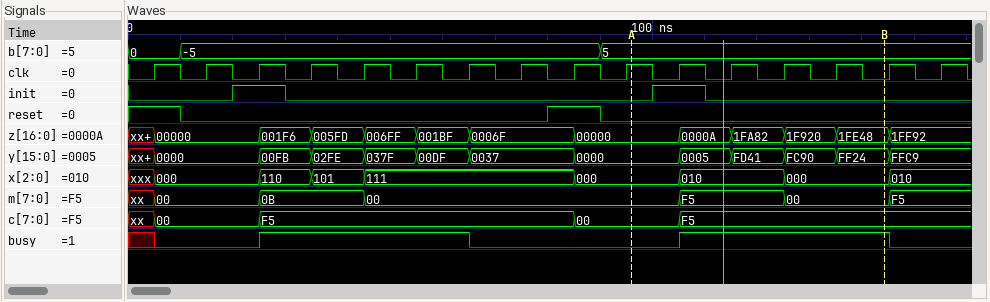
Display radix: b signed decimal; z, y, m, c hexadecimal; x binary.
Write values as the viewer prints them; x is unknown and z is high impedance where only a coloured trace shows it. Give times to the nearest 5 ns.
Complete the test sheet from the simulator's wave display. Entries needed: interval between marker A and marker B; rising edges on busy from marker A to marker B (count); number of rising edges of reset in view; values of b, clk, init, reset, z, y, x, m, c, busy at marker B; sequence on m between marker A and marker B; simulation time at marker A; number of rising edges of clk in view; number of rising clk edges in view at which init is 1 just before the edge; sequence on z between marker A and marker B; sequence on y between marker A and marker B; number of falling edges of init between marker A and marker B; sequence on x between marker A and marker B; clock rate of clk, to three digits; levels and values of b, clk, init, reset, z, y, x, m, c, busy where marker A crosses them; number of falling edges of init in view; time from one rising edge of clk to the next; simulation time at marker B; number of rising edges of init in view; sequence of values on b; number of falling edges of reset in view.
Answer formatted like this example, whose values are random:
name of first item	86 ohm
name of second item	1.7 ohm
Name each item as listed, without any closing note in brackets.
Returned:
interval between marker A and marker B	50 ns
rising edges on busy from marker A to marker B	1
number of rising edges of reset in view	1
values of b, clk, init, reset, z, y, x, m, c, busy at marker B	b=5, clk=0, init=0, reset=0, z=1FE48, y=FF24, x=000, m=00, c=F5, busy=1
sequence on m between marker A and marker B	00, F5, 00
simulation time at marker A	95 ns
number of rising edges of clk in view	16
number of rising clk edges in view at which init is 1 just before the edge	2
sequence on z between marker A and marker B	00000, 0000A, 1FA82, 1F920, 1FE48
sequence on y between marker A and marker B	0000, 0005, FD41, FC90, FF24
number of falling edges of init between marker A and marker B	1
sequence on x between marker A and marker B	000, 010, 000
clock rate of clk, to three digits	100 MHz
levels and values of b, clk, init, reset, z, y, x, m, c, busy where marker A crosses them	b=5, clk=1, init=0, reset=0, z=00000, y=0000, x=000, m=00, c=00, busy=0
number of falling edges of init in view	2
time from one rising edge of clk to the next	10 ns
simulation time at marker B	145 ns
number of rising edges of init in view	2
sequence of values on b	0, -5, 5
number of falling edges of reset in view	2
